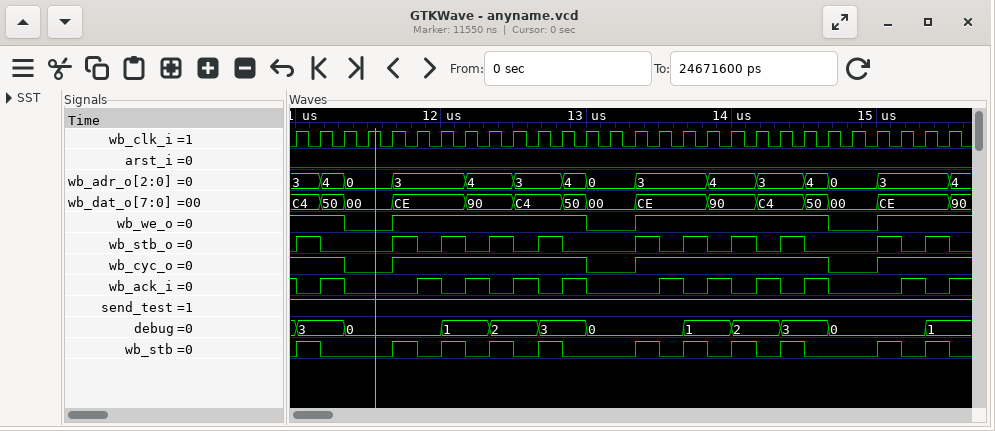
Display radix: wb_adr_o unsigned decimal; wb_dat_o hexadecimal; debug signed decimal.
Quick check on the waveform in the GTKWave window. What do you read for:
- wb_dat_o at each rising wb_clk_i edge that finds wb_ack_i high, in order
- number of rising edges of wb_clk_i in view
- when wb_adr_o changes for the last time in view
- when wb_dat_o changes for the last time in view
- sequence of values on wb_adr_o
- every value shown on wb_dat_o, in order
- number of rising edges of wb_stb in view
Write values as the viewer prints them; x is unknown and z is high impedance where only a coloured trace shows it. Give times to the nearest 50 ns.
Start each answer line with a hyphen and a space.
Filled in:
- C4, 50, CE, 90, C4, 50, CE, 90, C4, 50, CE
- 28
- 15500 ns
- 15500 ns
- 3, 4, 0, 3, 4, 3, 4, 0, 3, 4, 3, 4, 0, 3, 4
- C4, 50, 00, CE, 90, C4, 50, 00, CE, 90, C4, 50, 00, CE, 90
- 11
